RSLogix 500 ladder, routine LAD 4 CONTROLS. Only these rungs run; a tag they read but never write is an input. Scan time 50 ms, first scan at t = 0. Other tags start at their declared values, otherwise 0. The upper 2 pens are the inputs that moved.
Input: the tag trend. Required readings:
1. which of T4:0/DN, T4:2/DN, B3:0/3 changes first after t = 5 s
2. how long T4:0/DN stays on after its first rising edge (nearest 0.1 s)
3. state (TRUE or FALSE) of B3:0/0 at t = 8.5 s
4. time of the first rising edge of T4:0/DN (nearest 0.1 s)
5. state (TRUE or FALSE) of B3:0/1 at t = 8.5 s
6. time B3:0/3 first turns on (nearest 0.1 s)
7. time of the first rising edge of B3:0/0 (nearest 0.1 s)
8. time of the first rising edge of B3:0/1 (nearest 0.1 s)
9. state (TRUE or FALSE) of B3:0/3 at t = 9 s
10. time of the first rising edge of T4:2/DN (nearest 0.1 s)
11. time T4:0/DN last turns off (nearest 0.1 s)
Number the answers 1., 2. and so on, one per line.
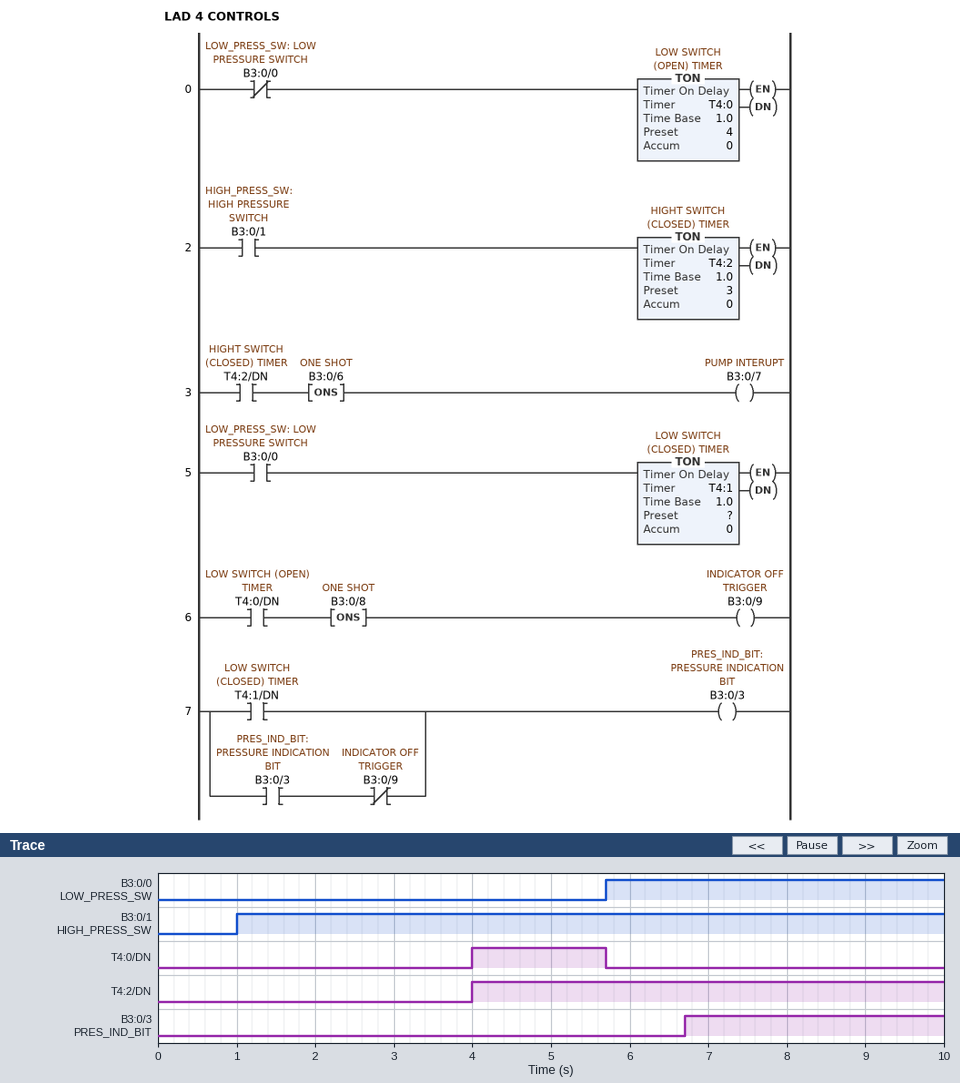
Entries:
1. T4:0/DN
2. 1.7 s
3. TRUE
4. 4.0 s
5. TRUE
6. 6.7 s
7. 5.7 s
8. 1.0 s
9. TRUE
10. 4.0 s
11. 5.7 s
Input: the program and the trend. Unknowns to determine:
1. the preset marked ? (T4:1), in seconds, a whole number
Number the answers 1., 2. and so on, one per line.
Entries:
1. 1 s
